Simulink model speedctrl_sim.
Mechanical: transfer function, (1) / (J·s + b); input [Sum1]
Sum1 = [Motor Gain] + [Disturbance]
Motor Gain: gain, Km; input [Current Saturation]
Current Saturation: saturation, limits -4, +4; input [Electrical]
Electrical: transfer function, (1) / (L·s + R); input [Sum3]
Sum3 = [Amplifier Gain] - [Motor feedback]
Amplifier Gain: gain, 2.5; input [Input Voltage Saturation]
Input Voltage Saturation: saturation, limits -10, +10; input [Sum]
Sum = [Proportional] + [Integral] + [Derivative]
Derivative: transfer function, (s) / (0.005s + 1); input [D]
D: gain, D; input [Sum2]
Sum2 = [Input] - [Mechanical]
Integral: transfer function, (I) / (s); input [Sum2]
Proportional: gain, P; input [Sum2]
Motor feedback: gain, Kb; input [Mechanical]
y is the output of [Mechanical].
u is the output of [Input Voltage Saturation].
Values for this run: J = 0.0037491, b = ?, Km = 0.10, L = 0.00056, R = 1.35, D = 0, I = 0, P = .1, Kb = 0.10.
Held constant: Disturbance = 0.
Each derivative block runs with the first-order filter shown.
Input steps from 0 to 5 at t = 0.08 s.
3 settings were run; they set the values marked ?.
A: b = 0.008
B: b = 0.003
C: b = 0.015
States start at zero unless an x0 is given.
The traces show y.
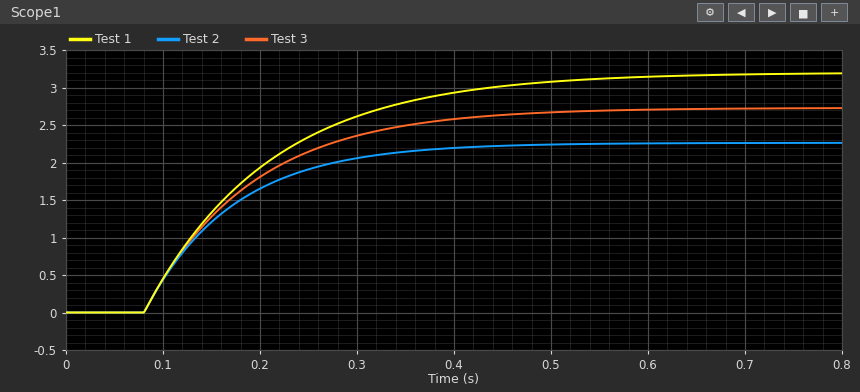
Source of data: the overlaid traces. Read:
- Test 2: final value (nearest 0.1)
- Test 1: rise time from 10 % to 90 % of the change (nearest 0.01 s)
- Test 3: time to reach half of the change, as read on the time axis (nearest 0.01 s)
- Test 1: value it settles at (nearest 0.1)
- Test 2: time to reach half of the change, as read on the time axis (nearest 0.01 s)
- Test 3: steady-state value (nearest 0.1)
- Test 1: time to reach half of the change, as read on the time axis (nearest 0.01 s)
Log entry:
2.3
0.28 s
0.16 s
3.2
0.14 s
2.7
0.17 s
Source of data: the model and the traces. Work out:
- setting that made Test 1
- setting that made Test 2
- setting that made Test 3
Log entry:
B
C
A
